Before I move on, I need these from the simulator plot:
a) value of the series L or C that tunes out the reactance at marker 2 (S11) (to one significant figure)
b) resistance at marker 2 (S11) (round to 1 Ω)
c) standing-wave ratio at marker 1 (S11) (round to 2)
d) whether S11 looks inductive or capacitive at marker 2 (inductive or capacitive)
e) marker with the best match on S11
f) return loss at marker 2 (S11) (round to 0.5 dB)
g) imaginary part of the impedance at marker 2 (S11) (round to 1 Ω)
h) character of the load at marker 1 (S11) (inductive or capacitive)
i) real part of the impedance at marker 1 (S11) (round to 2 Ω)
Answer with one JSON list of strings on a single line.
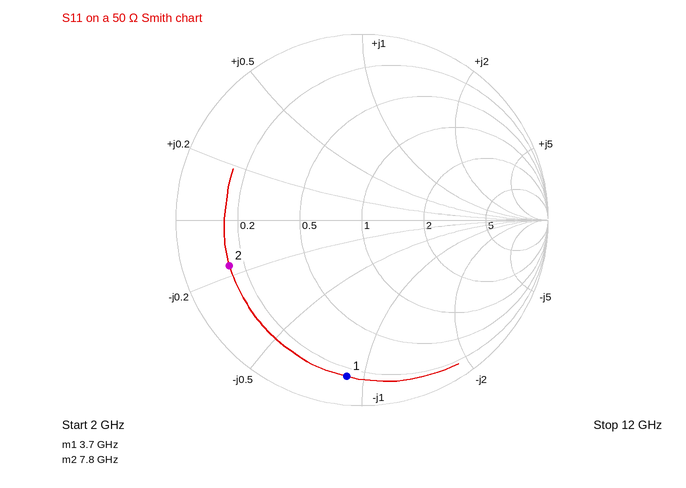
["200 pH", "7 Ω", "12", "capacitive", "marker 2", "2.5 dB", "-8 Ω", "capacitive", "8 Ω"]
